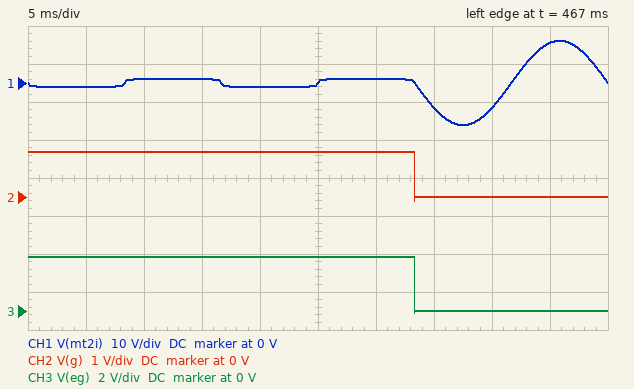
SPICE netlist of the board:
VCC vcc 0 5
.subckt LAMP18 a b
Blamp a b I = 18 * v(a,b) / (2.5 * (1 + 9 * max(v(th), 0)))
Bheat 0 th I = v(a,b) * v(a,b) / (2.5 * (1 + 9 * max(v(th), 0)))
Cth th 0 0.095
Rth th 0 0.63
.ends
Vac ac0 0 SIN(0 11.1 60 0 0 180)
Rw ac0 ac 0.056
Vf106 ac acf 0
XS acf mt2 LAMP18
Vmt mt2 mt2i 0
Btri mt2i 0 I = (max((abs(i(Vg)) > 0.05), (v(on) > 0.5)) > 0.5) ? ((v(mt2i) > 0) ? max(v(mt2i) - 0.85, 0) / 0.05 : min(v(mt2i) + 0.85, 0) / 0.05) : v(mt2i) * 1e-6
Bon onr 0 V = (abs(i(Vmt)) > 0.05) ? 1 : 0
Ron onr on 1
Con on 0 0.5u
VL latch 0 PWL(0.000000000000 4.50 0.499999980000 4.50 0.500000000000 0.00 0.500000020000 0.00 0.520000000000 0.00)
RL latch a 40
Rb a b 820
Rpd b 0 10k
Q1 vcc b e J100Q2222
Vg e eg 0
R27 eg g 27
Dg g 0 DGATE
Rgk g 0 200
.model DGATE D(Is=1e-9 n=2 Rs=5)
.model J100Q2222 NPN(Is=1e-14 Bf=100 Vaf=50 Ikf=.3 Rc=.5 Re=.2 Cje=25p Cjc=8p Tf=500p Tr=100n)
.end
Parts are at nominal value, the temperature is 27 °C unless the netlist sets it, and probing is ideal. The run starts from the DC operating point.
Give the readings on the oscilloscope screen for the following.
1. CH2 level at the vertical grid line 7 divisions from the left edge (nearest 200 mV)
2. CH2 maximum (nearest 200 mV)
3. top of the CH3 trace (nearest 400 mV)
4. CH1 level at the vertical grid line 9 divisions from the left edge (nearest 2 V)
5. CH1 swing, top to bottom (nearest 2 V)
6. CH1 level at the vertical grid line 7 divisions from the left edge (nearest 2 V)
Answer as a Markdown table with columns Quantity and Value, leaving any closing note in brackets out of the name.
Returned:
| Quantity | Value |
|---|---|
| CH2 level at the vertical grid line 7 divisions from the left edge | 0 V |
| CH2 maximum | 1.2 V |
| top of the CH3 trace | 2.8 V |
| CH1 level at the vertical grid line 9 divisions from the left edge | 10 V |
| CH1 swing, top to bottom | 22 V |
| CH1 level at the vertical grid line 7 divisions from the left edge | -6 V |
